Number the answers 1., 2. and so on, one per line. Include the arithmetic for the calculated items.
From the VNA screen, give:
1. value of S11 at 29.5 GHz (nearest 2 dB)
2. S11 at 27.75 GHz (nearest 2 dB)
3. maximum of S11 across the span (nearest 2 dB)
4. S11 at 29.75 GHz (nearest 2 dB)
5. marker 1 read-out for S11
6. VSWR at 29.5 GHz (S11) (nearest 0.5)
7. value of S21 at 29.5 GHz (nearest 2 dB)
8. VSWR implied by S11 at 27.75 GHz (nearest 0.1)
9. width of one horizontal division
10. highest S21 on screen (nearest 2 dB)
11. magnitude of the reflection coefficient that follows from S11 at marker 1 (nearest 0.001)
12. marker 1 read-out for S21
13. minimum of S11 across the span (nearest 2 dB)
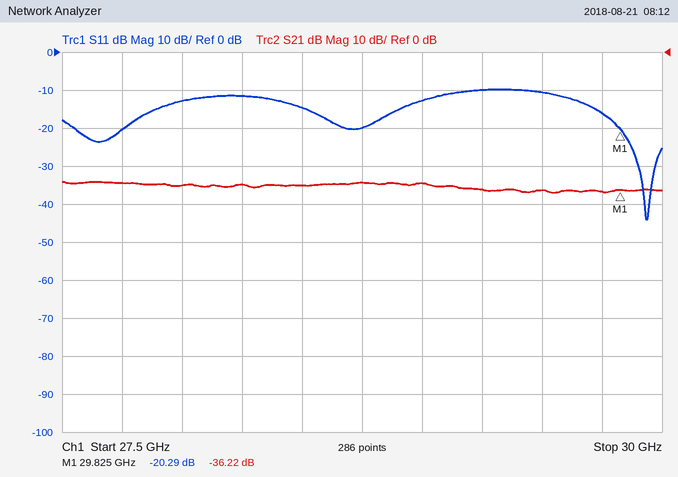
1. -10 dB
2. -20 dB
3. -10 dB
4. -16 dB
5. -20.29 dB
6. |Γ| = 10^(-10/20) = 0.3162; VSWR = (1 + 0.3162)/(1 − 0.3162) ≈ 1.92, so 2.0 to the nearest 0.5
7. -36 dB
8. |Γ| = 10^(-20/20) = 0.1000; VSWR = (1 + 0.1000)/(1 − 0.1000) ≈ 1.2
9. 250 MHz
10. -34 dB
11. 10^(-20.29/20) ≈ 0.097
12. -36.22 dB
13. -44 dB
